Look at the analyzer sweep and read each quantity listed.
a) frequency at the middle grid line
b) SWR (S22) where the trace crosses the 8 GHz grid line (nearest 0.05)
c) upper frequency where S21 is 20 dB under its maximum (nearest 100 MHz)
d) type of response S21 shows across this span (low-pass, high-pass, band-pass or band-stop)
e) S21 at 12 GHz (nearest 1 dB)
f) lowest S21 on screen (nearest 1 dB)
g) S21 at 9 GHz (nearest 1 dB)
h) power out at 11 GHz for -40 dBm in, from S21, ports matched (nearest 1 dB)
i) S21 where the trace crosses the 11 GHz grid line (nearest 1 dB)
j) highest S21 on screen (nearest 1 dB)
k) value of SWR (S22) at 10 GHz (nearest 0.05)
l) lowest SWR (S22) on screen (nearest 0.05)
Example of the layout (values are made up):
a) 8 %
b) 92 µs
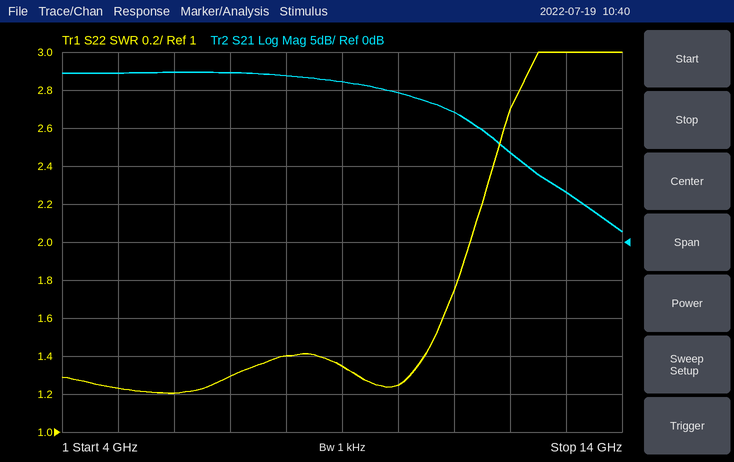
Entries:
a) 9 GHz
b) 1.40
c) 13.8 GHz
d) low-pass
e) 12 dB
f) 1 dB
g) 21 dB
h) -23 dBm
i) 17 dB
j) 22 dB
k) 1.25
l) 1.20
